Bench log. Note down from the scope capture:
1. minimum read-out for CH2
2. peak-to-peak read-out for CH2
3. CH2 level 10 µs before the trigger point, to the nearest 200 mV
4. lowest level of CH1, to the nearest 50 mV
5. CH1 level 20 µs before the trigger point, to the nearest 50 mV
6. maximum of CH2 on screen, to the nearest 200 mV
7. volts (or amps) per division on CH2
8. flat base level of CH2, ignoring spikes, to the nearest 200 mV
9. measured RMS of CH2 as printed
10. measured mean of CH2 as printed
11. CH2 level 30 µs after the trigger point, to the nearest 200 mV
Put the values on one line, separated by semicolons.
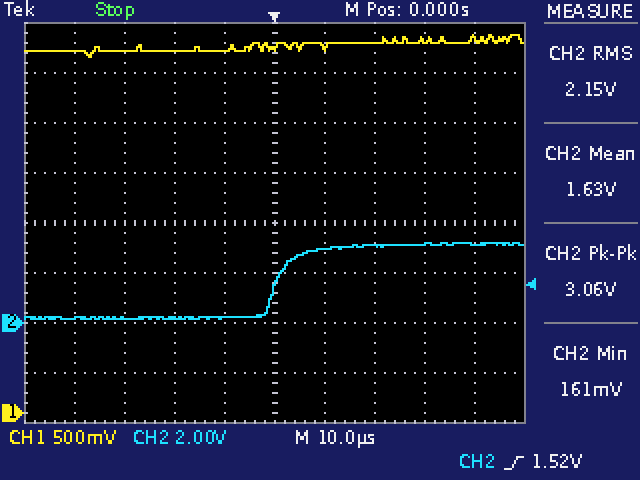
161 mV; 3.06 V; 200 mV; 3.55 V; 3.60 V; 3.2 V; 2 V; 200 mV; 2.15 V; 1.63 V; 3.2 V
